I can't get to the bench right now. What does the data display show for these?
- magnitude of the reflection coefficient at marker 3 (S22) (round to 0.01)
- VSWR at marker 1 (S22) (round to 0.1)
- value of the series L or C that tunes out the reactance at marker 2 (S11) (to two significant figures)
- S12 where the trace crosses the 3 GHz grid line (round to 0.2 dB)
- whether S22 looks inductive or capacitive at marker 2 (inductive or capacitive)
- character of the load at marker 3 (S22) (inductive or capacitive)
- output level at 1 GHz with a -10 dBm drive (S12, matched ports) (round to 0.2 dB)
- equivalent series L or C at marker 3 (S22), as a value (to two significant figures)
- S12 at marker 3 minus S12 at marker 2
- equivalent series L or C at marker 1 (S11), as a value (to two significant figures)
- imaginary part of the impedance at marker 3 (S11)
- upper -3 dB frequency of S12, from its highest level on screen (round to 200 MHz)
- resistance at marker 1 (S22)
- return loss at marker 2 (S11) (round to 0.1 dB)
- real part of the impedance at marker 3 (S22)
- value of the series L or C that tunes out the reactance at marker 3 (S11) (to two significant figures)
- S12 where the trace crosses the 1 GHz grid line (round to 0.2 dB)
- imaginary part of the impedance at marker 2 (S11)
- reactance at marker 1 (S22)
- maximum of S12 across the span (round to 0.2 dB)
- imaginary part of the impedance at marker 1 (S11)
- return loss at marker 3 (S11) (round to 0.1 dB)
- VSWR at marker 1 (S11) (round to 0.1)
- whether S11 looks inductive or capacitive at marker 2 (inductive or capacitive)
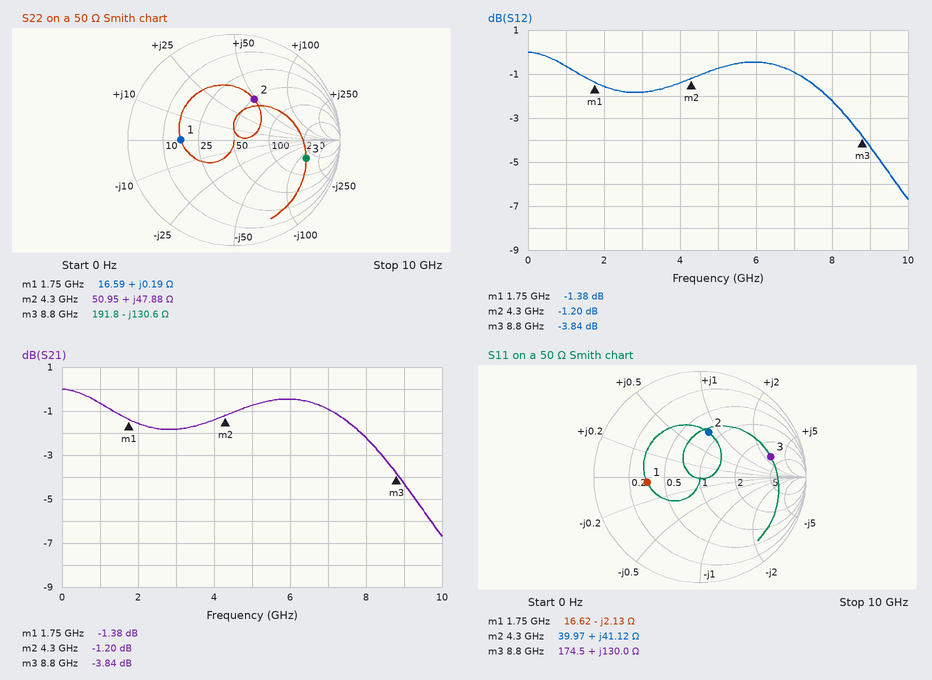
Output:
0.70
3.0
900 fF
-1.8 dB
inductive
capacitive
-10.6 dBm
140 fF
-2.64 dB
43 pF
+130.0 Ω
8.4 GHz
16.59 Ω
7.4 dB
191.8 Ω
140 fF
-0.6 dB
+41.12 Ω
+0.19 Ω
0.0 dB
-2.13 Ω
3.2 dB
3.0
inductive
